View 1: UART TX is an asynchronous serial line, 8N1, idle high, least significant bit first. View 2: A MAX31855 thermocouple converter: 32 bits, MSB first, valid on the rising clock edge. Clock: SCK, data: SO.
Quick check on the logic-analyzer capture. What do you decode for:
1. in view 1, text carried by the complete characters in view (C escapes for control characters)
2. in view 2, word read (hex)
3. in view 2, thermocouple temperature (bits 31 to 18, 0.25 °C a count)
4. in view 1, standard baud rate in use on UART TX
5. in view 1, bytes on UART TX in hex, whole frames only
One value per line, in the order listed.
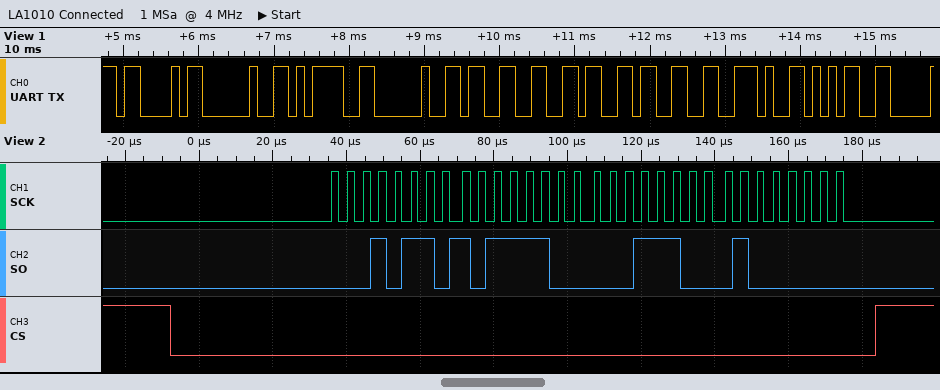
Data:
"C = 363.5"
0x16BC1C40
363.75 °C
9600 baud
43 20 3D 20 33 36 33 2E 35
